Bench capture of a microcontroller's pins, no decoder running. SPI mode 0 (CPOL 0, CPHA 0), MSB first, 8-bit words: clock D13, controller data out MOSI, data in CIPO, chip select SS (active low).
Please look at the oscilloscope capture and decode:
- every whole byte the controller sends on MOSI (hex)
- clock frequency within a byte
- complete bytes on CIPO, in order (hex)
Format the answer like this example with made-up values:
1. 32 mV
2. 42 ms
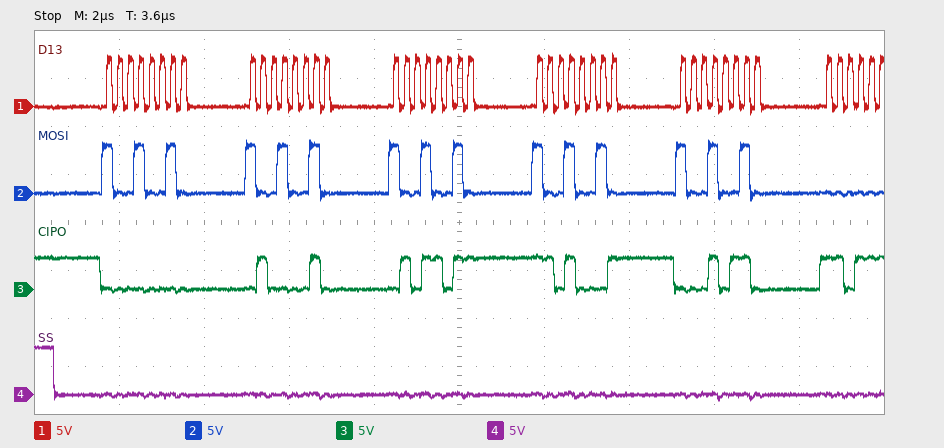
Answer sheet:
1. 92 92 92 92 92
2. 4 MHz
3. 00 42 5B D1 16
